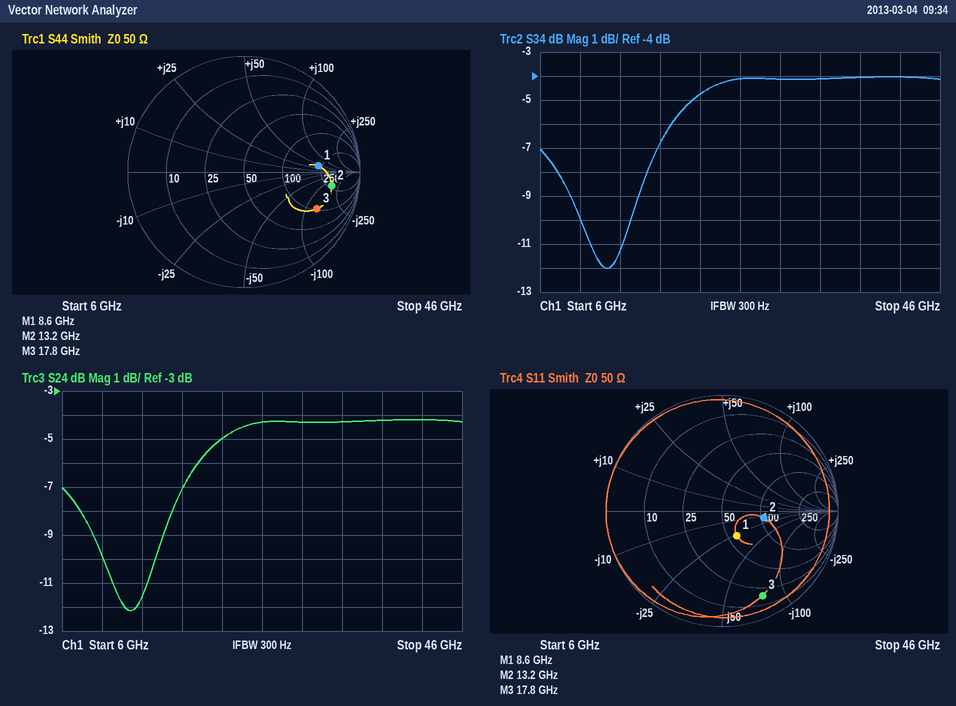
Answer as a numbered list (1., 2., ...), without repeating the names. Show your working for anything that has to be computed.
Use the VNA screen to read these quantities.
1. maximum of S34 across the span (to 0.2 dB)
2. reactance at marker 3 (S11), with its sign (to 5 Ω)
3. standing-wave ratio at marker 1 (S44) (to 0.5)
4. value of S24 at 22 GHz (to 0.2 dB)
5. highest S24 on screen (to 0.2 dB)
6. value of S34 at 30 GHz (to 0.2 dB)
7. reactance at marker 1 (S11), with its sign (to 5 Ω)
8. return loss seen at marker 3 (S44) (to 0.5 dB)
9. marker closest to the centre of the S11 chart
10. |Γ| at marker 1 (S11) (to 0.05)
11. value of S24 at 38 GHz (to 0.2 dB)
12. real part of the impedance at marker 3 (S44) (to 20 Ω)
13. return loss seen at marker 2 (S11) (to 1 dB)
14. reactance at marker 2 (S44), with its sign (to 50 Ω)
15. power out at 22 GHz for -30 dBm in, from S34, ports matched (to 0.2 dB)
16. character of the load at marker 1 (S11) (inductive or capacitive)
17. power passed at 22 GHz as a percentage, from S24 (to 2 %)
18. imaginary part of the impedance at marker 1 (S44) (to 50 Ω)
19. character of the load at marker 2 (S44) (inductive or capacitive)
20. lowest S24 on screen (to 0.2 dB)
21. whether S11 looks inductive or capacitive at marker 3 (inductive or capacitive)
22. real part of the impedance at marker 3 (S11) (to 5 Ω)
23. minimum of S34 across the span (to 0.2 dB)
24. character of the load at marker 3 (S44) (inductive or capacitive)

1. -4.0 dB
2. -75 Ω
3. 4.5
4. -5.0 dB
5. -4.2 dB
6. -4.2 dB
7. -25 Ω
8. 3.0 dB
9. marker 1
10. 0.25
11. -4.2 dB
12. 100 Ω
13. 9 dB
14. -150 Ω
15. -30 dBm + (-4.8 dB) = -34.8 dBm
16. capacitive
17. 10^(-5/10) ≈ 32 %
18. +50 Ω
19. capacitive
20. -12.2 dB
21. capacitive
22. 20 Ω
23. -12.0 dB
24. capacitive
